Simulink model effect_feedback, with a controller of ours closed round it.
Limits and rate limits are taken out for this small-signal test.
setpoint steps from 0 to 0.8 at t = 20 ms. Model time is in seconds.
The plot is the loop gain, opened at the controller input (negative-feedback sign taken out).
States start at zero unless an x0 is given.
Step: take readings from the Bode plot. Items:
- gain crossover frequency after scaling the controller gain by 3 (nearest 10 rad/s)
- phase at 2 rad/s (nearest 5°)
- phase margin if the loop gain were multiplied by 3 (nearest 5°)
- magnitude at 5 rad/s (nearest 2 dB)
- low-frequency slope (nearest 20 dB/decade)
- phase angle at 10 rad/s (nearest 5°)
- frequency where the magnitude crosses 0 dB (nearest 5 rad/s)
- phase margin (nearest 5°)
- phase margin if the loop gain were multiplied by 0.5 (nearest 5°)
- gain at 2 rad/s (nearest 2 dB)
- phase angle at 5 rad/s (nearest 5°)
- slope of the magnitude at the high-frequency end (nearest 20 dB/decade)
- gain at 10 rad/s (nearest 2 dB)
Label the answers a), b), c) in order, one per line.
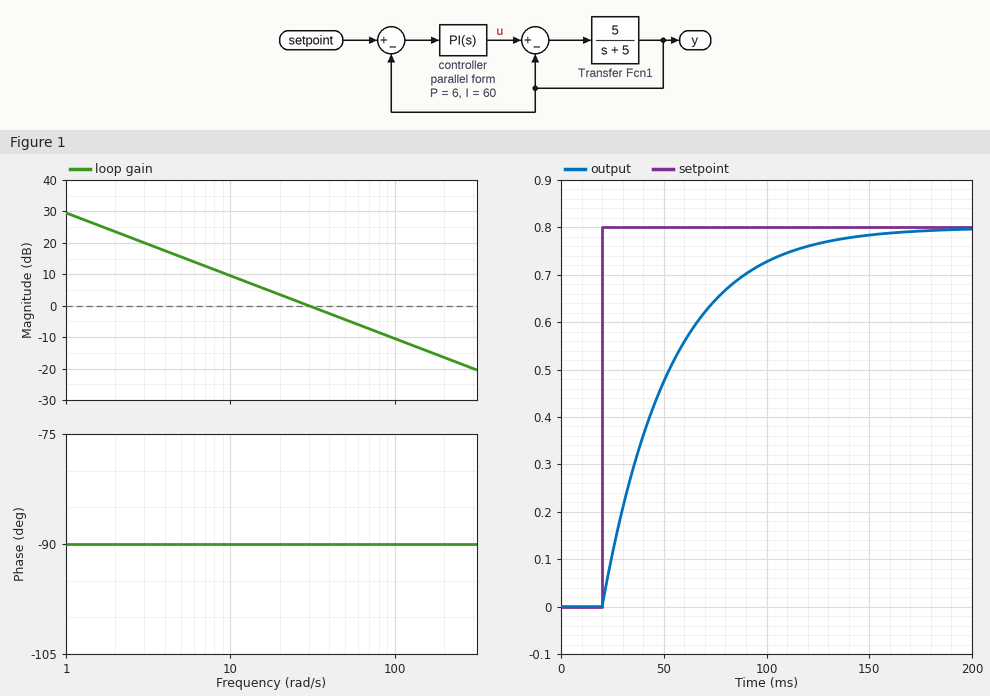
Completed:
a) 90 rad/s
b) -90°
c) 90°
d) 16 dB
e) -20 dB/decade
f) -90°
g) 30 rad/s
h) 90°
i) 90°
j) 24 dB
k) -90°
l) -20 dB/decade
m) 10 dB
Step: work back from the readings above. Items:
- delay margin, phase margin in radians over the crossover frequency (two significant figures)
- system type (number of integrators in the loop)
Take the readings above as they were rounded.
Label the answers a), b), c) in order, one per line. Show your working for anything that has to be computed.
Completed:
a) 90 × π / 180 / 30 = 0.052 s
b) 1
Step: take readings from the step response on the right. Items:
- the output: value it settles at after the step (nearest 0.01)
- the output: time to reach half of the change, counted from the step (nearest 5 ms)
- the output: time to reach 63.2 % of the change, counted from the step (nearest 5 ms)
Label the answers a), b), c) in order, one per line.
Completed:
a) 0.80
b) 25 ms
c) 35 ms
